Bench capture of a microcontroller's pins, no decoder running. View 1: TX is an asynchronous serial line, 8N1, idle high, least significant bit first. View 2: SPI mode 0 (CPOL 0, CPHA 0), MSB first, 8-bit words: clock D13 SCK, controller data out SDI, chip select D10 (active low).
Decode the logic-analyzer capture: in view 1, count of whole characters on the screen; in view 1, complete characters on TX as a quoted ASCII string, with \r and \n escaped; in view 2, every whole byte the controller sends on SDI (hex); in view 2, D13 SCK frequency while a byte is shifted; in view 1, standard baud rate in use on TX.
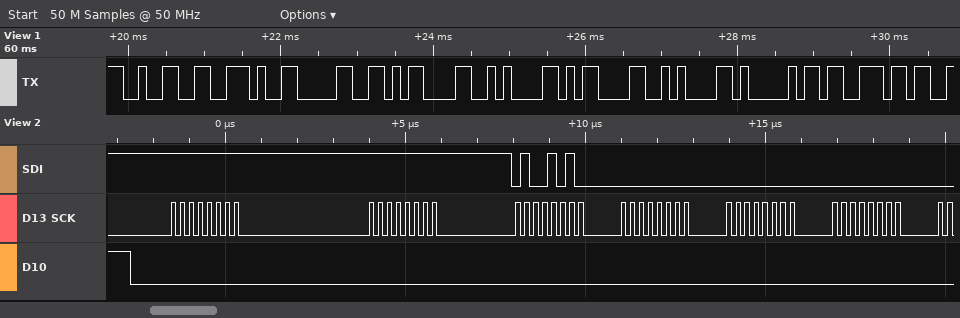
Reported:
9
"2.0\r\n\r\nAs"
FF FF 4A 00 00 00
4 MHz
9600 baud
